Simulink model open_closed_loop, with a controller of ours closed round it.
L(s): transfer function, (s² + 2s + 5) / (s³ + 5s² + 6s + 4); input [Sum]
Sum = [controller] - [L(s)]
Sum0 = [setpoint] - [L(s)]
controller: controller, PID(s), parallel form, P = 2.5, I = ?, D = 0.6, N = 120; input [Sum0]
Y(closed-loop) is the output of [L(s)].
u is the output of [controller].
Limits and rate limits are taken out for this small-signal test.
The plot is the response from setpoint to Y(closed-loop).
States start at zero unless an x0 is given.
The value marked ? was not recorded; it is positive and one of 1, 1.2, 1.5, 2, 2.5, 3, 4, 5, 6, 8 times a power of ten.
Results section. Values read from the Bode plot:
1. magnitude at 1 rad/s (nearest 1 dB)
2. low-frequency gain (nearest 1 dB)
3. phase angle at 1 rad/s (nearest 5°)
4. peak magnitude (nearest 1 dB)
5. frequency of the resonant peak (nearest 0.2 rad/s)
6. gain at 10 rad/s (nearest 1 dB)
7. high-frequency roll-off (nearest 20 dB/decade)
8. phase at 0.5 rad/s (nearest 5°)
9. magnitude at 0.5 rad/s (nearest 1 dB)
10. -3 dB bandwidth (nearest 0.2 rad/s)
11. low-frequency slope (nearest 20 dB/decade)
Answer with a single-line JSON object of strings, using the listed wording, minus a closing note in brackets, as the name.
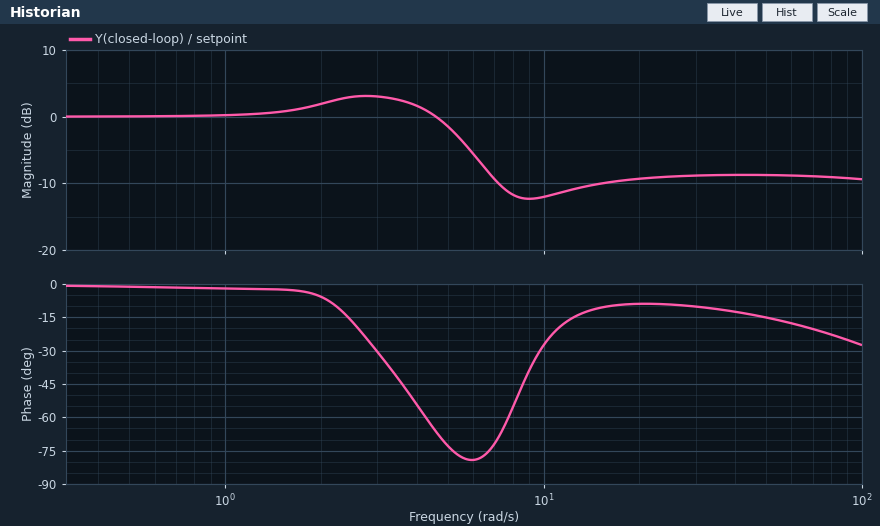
{"magnitude at 1 rad/s": "0 dB", "low-frequency gain": "0 dB", "phase angle at 1 rad/s": "0°", "peak magnitude": "3 dB", "frequency of the resonant peak": "2.8 rad/s", "gain at 10 rad/s": "-12 dB", "high-frequency roll-off": "0 dB/decade", "phase at 0.5 rad/s": "0°", "magnitude at 0.5 rad/s": "0 dB", "-3 dB bandwidth": "5.4 rad/s", "low-frequency slope": "0 dB/decade"}
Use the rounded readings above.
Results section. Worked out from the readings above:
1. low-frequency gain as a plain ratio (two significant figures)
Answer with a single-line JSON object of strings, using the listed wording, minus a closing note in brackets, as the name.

{"low-frequency gain as a plain ratio": "1.0"}
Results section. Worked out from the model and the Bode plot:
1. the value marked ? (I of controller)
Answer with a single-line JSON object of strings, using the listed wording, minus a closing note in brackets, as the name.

{"the value marked ?": "40"}
